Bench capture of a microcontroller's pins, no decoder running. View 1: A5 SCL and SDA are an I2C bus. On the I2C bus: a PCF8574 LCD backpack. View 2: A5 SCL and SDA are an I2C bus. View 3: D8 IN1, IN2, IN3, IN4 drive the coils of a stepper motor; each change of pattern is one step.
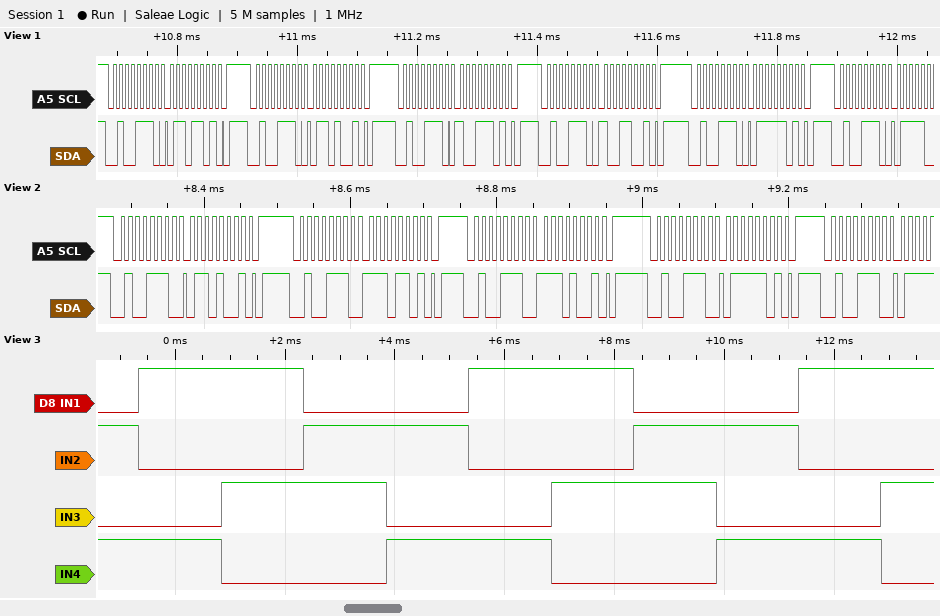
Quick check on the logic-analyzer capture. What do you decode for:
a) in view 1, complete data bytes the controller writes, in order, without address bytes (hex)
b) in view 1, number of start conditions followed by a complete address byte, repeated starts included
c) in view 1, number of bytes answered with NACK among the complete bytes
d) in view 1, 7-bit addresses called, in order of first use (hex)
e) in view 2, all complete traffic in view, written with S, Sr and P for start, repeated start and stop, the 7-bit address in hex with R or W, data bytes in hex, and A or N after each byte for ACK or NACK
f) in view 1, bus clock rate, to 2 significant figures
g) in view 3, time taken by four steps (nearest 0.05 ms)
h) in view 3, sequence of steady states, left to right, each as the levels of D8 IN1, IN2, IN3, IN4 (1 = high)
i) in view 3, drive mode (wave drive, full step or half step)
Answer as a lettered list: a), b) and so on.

a) 6D 69 9D 99 7D
b) 6
c) 0
d) 0x27
e) S 27W A 69 A P S 27W A ED A P S 27W A E9 A P S 27W A 7D A P S 27W A
f) 100 kHz
g) 6.00 ms
h) 0101 1001 1010 0110 0101 1001 1010 0110 0101 1001 1010
i) full step
